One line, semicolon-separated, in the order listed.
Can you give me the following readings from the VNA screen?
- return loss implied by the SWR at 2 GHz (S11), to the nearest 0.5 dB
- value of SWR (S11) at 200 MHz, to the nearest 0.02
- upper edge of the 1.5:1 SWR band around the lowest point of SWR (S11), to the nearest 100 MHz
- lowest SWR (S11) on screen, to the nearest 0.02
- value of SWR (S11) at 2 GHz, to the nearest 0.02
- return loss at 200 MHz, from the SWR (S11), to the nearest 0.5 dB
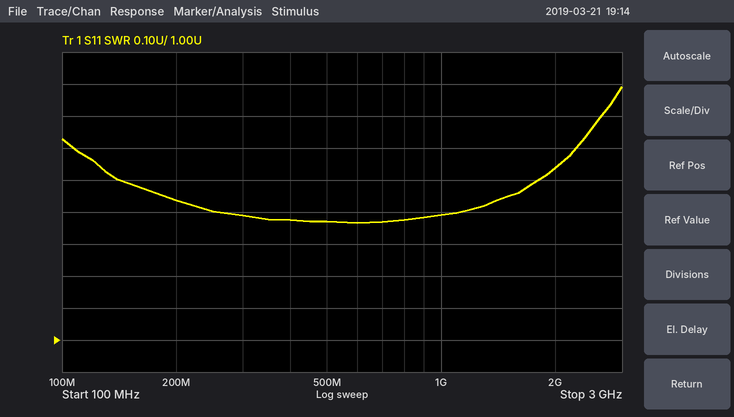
13.5 dB; 1.44; 1.8 GHz; 1.36; 1.54; 15.0 dB
